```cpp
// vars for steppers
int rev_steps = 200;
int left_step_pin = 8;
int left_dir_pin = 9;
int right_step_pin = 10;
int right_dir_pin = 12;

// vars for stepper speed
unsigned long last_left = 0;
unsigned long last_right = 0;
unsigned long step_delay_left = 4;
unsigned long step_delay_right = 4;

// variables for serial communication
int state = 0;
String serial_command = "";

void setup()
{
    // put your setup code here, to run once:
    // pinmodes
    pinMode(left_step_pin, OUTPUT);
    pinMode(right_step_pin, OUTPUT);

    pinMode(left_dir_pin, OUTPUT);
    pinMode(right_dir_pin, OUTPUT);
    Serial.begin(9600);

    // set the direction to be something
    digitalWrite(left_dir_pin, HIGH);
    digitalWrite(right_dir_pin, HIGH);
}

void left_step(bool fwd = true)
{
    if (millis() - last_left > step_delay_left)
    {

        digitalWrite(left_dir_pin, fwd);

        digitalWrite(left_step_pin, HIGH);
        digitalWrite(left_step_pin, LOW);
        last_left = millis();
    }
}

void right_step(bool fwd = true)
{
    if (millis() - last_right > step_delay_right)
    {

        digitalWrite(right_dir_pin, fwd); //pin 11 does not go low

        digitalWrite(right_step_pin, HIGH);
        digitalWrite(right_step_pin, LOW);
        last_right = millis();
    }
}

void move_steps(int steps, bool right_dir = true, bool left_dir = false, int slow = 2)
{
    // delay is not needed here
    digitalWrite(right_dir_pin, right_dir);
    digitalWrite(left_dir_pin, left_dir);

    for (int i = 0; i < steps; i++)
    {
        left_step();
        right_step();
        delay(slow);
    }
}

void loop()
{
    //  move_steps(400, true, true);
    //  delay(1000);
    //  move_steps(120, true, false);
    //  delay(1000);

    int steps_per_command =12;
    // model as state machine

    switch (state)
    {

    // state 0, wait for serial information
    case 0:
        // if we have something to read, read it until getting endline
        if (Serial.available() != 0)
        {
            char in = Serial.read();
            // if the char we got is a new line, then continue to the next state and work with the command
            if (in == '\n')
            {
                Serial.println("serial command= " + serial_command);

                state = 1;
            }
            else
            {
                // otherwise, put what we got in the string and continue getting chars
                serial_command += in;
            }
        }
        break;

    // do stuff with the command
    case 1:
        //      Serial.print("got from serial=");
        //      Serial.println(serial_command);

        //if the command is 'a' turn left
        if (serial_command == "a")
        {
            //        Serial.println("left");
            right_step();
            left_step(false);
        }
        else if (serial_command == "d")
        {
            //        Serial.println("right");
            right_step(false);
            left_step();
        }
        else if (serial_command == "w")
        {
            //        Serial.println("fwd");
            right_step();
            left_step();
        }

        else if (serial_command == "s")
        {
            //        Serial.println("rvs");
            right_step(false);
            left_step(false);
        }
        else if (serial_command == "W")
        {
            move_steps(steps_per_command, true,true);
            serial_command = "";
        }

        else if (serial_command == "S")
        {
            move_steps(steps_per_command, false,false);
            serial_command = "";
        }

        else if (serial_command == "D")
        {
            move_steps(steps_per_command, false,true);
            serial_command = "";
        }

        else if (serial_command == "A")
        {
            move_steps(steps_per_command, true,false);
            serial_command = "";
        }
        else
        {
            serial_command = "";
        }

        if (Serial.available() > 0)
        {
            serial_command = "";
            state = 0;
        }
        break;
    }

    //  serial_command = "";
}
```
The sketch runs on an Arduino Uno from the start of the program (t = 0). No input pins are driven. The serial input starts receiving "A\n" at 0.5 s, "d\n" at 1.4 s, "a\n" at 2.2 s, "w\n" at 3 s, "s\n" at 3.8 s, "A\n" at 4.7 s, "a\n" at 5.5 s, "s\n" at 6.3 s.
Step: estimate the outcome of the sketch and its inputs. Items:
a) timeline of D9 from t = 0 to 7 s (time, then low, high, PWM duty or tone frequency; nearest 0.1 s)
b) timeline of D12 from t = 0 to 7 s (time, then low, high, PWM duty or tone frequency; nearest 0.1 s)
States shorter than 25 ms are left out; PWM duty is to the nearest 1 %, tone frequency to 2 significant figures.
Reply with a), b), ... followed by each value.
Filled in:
a) 0 s high; 2.2 s low; 3 s high; 3.8 s low; 4.7 s high; 5.5 s low
b) 0 s high; 1.4 s low; 2.2 s high; 3.8 s low; 4.7 s high; 6.3 s low
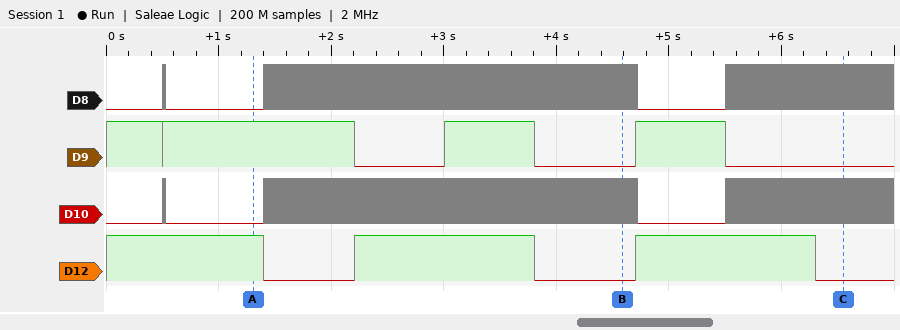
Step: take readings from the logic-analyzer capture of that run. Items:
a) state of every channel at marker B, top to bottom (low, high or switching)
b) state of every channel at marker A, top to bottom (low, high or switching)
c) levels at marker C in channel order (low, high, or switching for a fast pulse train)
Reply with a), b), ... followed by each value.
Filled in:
a) D8 switching, D9 low, D10 switching, D12 low
b) D8 low, D9 high, D10 low, D12 high
c) D8 switching, D9 low, D10 switching, D12 low
